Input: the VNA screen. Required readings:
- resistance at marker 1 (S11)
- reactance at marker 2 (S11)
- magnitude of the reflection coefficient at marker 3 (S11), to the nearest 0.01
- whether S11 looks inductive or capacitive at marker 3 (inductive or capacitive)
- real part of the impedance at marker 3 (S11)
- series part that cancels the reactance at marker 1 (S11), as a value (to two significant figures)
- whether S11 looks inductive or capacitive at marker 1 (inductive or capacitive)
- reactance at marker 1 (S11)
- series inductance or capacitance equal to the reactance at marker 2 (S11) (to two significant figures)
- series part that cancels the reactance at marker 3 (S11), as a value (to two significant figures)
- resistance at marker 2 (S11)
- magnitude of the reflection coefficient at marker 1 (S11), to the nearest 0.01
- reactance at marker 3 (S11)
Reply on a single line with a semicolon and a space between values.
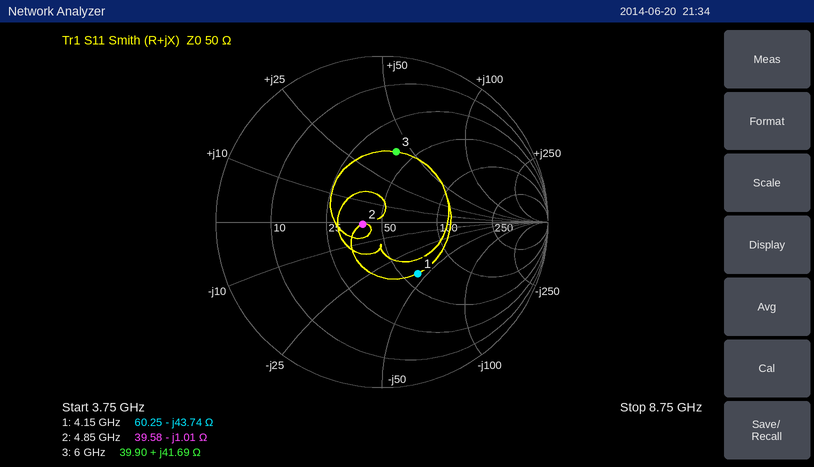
60.25 Ω; -1.01 Ω; 0.43; inductive; 39.90 Ω; 1.7 nH; capacitive; -43.74 Ω; 32 pF; 640 fF; 39.58 Ω; 0.38; +41.69 Ω
